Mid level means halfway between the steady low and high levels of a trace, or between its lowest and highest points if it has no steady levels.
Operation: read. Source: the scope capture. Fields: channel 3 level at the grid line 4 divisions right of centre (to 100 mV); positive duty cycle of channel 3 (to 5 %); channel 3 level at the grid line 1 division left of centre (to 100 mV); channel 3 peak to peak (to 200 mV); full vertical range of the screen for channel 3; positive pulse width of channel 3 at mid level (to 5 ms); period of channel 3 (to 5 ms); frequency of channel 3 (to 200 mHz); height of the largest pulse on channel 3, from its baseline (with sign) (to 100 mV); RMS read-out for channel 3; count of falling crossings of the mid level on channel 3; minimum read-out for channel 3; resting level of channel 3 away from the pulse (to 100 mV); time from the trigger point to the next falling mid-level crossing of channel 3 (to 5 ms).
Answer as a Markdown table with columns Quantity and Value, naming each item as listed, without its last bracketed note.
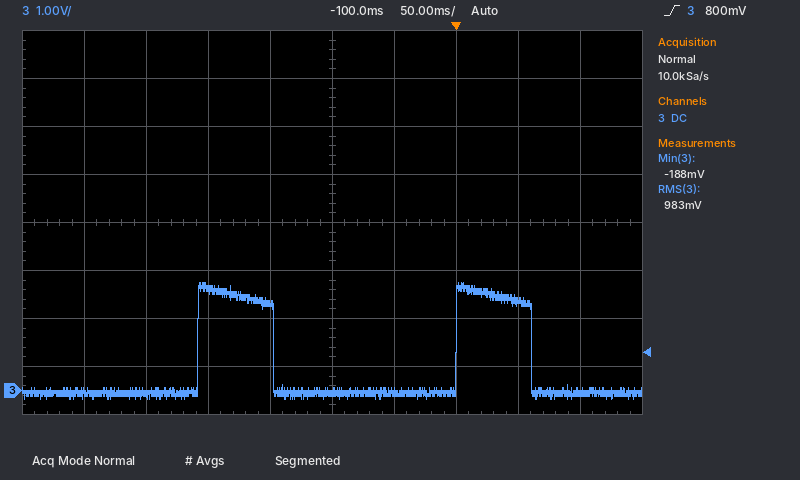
| Quantity | Value |
|---|---|
| channel 3 level at the grid line 4 divisions right of centre | 0.0 V |
| positive duty cycle of channel 3 | 30 % |
| channel 3 level at the grid line 1 division left of centre | 1.8 V |
| channel 3 peak to peak | 2.4 V |
| full vertical range of the screen for channel 3 | 8 V |
| positive pulse width of channel 3 at mid level | 60 ms |
| period of channel 3 | 210 ms |
| frequency of channel 3 | 4.8 Hz |
| height of the largest pulse on channel 3, from its baseline (with sign) | +2.3 V |
| RMS read-out for channel 3 | 983 mV |
| count of falling crossings of the mid level on channel 3 | 2 |
| minimum read-out for channel 3 | -188 mV |
| resting level of channel 3 away from the pulse | -100 mV |
| time from the trigger point to the next falling mid-level crossing of channel 3 | 60 ms |
